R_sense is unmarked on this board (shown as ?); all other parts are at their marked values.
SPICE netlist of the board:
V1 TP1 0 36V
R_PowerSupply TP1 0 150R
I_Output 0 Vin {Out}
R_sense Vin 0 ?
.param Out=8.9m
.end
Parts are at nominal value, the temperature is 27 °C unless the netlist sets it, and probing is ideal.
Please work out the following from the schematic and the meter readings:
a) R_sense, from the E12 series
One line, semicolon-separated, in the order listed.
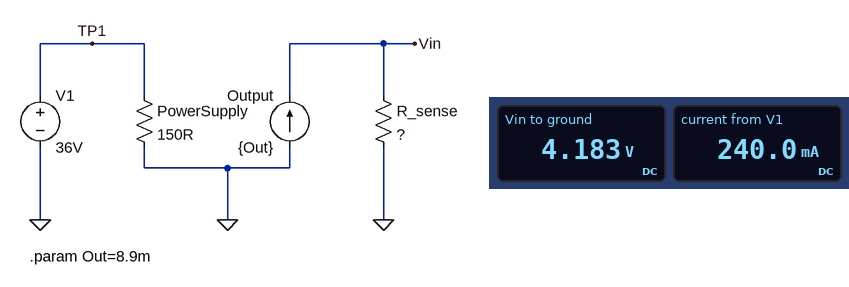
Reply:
470 Ω
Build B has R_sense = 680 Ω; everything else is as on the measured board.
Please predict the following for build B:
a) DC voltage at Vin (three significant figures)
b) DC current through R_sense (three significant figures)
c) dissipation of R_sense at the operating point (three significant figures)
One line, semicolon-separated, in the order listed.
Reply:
6.05 V; 8.90 mA; 53.9 mW
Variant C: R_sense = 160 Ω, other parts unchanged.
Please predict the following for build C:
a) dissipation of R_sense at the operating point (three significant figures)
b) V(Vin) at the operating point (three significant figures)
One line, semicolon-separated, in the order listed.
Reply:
12.7 mW; 1.42 V
